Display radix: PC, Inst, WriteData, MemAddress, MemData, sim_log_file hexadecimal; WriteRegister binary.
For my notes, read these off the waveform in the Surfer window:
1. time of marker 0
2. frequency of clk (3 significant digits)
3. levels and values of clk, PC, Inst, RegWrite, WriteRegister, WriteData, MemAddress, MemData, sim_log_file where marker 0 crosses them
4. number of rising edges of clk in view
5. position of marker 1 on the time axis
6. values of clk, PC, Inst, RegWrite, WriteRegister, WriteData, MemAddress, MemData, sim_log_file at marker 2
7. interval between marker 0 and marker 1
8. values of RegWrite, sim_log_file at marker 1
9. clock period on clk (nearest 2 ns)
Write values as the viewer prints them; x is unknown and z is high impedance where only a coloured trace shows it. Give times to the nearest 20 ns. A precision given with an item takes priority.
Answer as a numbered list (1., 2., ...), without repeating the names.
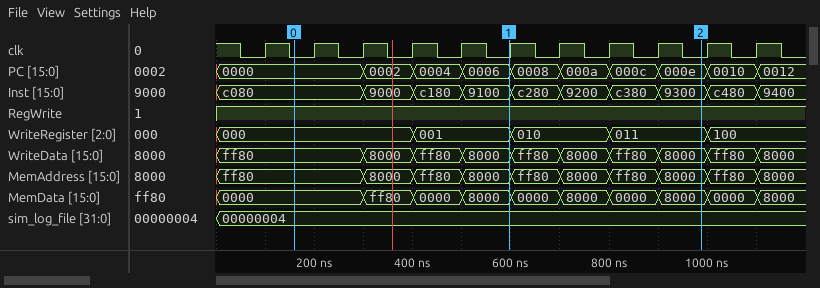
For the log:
1. 160 ns
2. 10.0 MHz
3. clk=0, PC=0000, Inst=c080, RegWrite=1, WriteRegister=000, WriteData=ff80, MemAddress=ff80, MemData=0000, sim_log_file=00000004
4. 11
5. 600 ns
6. clk=0, PC=000e, Inst=9300, RegWrite=1, WriteRegister=011, WriteData=8000, MemAddress=8000, MemData=8000, sim_log_file=00000004
7. 440 ns
8. RegWrite=1, sim_log_file=00000004
9. 100 ns
